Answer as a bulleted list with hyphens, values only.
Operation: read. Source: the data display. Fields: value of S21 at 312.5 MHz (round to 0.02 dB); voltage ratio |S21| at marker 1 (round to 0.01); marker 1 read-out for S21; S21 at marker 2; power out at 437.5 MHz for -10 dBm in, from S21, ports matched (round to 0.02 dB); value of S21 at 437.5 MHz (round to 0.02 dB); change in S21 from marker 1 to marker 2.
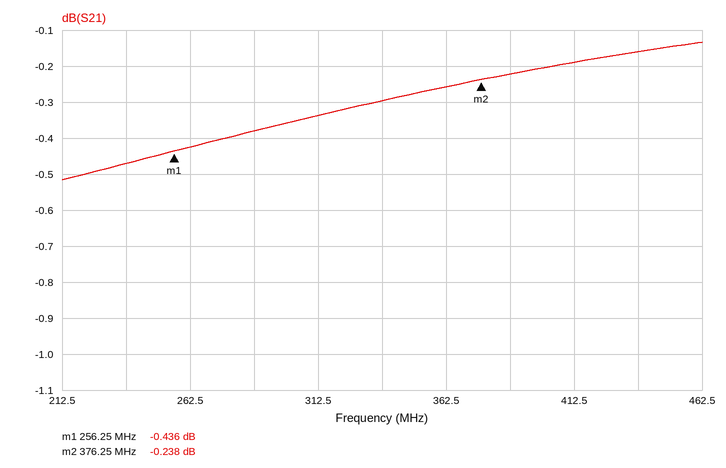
- -0.34 dB
- 0.95
- -0.436 dB
- -0.238 dB
- -10.16 dBm
- -0.16 dB
- 0.198 dB
